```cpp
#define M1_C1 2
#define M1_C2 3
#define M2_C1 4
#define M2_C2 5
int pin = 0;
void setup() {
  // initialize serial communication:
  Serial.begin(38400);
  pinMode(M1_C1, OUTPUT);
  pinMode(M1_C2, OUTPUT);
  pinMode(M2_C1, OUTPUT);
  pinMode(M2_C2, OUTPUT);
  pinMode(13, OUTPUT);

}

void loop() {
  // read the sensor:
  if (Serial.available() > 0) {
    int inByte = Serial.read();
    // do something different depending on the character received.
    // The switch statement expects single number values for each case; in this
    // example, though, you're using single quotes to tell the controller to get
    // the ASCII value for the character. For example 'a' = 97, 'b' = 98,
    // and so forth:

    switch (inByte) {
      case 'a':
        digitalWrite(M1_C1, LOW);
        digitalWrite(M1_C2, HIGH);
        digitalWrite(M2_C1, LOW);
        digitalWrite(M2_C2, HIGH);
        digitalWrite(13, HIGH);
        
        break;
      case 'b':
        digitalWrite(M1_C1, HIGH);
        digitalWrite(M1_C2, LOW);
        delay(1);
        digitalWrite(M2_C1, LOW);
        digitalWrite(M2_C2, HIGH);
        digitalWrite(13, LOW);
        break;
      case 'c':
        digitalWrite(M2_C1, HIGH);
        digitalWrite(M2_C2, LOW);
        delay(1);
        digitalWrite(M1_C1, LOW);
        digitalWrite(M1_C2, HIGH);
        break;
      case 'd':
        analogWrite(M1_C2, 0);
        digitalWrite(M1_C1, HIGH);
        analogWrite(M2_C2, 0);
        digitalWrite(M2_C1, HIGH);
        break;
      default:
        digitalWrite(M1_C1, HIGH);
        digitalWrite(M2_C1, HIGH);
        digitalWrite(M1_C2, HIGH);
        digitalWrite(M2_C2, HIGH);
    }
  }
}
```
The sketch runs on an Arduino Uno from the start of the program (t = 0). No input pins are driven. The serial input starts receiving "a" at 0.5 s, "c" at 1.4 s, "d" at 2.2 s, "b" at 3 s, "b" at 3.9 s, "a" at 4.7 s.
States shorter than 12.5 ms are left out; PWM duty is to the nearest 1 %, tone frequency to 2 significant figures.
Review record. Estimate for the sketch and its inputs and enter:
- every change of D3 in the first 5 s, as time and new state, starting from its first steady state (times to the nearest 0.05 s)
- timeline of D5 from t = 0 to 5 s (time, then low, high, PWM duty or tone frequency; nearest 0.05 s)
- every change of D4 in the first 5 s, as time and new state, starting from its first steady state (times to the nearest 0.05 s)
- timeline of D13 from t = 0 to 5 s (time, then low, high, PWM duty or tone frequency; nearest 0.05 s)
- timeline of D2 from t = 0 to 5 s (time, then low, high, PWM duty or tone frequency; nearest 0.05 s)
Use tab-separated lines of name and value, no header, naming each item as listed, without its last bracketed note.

every change of D3 in the first 5 s, as time and new state, starting from its first steady state	0 s low; 0.5 s high; 2.2 s low; 4.7 s high
timeline of D5 from t = 0 to 5 s	0 s low; 0.5 s high; 1.4 s low; 3 s high
every change of D4 in the first 5 s, as time and new state, starting from its first steady state	0 s low; 1.4 s high; 3 s low
timeline of D13 from t = 0 to 5 s	0 s low; 0.5 s high; 3 s low; 4.7 s high
timeline of D2 from t = 0 to 5 s	0 s low; 2.2 s high; 4.7 s low
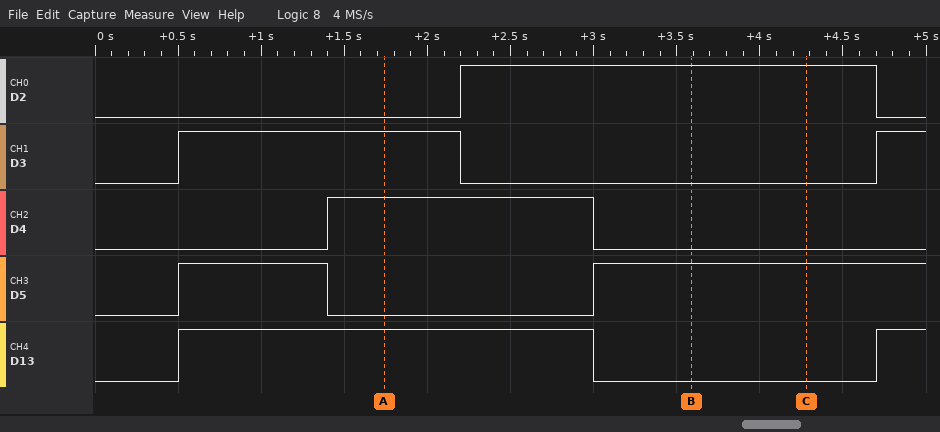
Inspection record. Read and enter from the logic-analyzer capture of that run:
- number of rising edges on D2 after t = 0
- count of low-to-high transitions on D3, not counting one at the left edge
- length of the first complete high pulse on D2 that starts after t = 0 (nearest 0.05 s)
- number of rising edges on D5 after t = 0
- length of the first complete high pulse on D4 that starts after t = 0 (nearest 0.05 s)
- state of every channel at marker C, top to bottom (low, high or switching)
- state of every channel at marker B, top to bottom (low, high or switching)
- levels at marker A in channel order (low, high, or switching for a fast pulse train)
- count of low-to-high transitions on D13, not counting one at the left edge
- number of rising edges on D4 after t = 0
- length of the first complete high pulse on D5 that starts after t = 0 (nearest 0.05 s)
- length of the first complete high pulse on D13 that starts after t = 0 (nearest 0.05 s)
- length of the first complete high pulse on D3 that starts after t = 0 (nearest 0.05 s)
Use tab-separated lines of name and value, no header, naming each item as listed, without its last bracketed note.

number of rising edges on D2 after t = 0	1
count of low-to-high transitions on D3, not counting one at the left edge	2
length of the first complete high pulse on D2 that starts after t = 0	2.50 s
number of rising edges on D5 after t = 0	2
length of the first complete high pulse on D4 that starts after t = 0	1.60 s
state of every channel at marker C, top to bottom	D2 high, D3 low, D4 low, D5 high, D13 low
state of every channel at marker B, top to bottom	D2 high, D3 low, D4 low, D5 high, D13 low
levels at marker A in channel order	D2 low, D3 high, D4 high, D5 low, D13 high
count of low-to-high transitions on D13, not counting one at the left edge	2
number of rising edges on D4 after t = 0	1
length of the first complete high pulse on D5 that starts after t = 0	0.90 s
length of the first complete high pulse on D13 that starts after t = 0	2.50 s
length of the first complete high pulse on D3 that starts after t = 0	1.70 s
